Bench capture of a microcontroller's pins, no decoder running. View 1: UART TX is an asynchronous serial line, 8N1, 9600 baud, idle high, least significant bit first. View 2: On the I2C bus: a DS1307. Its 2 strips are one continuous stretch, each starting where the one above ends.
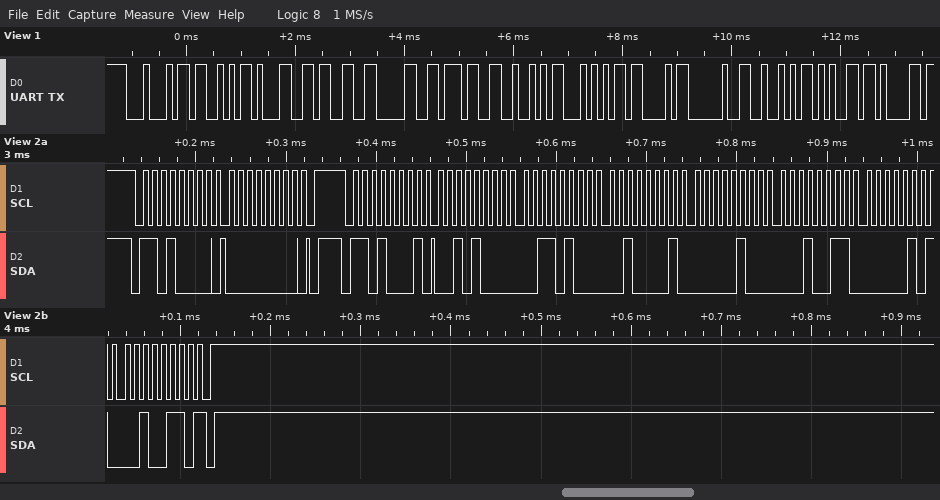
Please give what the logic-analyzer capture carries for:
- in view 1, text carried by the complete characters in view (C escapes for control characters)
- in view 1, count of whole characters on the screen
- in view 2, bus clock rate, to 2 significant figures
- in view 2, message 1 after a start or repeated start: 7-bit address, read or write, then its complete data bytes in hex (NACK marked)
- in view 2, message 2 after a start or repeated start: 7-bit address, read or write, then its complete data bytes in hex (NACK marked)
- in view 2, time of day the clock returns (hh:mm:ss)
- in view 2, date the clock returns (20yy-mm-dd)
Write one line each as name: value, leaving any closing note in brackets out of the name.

in view 1, text carried by the complete characters in view: "DS1307RTC Rea"
in view 1, count of whole characters on the screen: 13
in view 2, bus clock rate, to 2 significant figures: 100 kHz
in view 2, message 1 after a start or repeated start: 7-bit address, read or write, then its complete data bytes in hex: 0x68 write: 00
in view 2, message 2 after a start or repeated start: 7-bit address, read or write, then its complete data bytes in hex: 0x68 read: 28 34 21 04 13 05 26 NACK
in view 2, time of day the clock returns: 21:34:28
in view 2, date the clock returns: 2026-05-13
